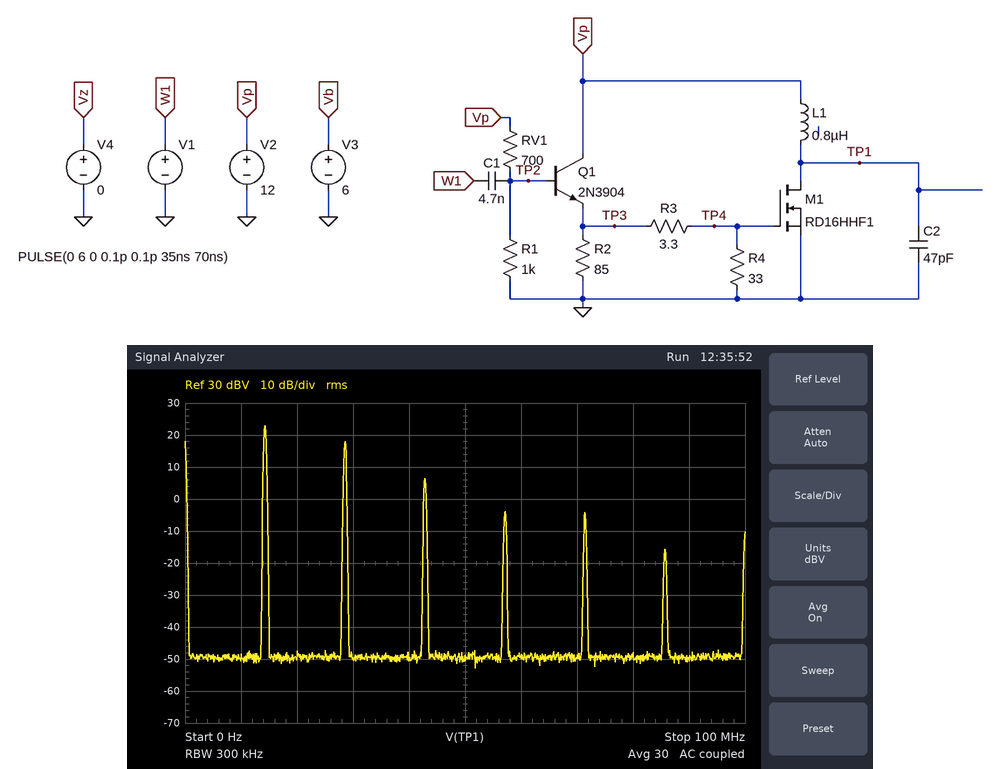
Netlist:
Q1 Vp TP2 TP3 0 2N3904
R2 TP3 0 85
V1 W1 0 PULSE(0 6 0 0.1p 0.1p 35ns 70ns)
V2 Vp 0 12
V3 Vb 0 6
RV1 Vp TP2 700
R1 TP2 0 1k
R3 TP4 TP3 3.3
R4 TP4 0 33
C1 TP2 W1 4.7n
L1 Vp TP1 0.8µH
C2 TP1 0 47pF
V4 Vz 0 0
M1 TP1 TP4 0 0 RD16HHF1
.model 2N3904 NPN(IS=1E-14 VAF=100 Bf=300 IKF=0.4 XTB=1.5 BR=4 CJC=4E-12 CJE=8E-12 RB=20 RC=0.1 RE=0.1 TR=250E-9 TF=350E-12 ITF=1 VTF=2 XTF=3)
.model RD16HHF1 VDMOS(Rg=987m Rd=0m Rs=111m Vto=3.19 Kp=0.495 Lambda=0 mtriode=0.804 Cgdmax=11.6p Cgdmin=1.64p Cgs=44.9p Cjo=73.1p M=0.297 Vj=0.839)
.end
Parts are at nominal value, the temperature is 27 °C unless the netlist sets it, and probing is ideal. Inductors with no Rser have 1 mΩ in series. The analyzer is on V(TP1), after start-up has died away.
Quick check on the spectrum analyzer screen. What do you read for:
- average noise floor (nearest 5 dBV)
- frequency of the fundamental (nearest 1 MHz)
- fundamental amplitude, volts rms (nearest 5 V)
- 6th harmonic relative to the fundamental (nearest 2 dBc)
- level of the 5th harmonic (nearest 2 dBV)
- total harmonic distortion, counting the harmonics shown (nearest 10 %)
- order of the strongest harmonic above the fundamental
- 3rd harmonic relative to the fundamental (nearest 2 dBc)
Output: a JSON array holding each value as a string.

["-50 dBV", "14 MHz", "15 V", "-38 dBc", "-4 dBV", "60 %", "2", "-16 dBc"]
